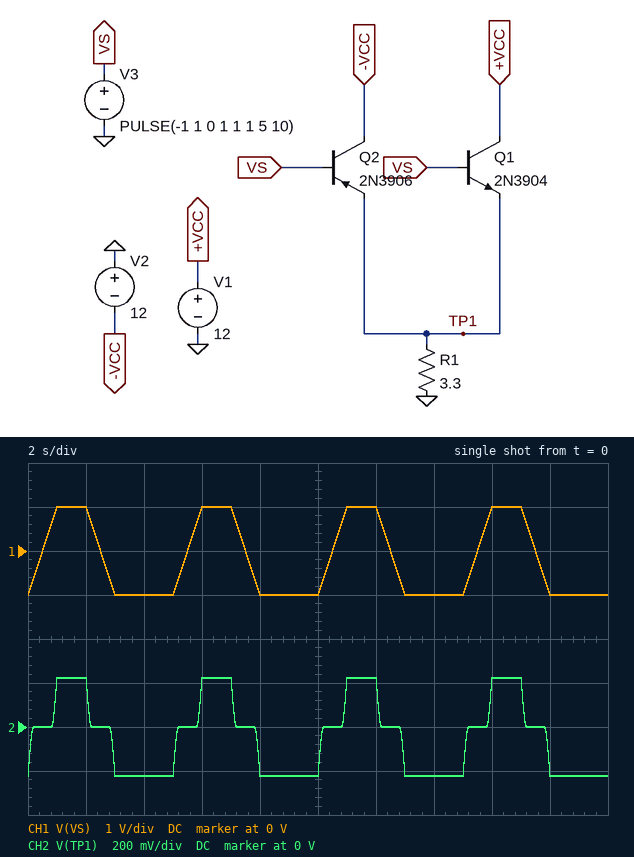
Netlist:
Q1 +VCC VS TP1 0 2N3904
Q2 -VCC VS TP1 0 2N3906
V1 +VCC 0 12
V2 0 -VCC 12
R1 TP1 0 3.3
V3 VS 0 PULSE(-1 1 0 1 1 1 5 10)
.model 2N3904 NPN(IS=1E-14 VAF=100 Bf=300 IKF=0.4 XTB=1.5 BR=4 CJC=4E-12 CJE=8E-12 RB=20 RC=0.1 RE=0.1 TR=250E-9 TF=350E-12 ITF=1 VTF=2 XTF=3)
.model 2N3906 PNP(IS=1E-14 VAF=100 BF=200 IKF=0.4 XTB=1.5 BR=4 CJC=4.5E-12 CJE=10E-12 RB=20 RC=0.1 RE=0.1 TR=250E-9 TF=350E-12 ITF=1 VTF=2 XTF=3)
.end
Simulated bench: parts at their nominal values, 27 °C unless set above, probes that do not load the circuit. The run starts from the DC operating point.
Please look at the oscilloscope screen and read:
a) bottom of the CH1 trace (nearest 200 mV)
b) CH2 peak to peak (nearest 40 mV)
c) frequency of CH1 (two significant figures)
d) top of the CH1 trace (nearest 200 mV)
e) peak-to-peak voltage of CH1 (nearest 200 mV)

-1.0 V
440 mV
200 mHz
1.0 V
2.0 V
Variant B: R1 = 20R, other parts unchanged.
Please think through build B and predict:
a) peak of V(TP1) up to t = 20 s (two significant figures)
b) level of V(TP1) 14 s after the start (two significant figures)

280 mV
-280 mV
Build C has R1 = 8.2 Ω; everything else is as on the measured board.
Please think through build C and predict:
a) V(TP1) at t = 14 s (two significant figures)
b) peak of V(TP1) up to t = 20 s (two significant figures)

-250 mV
250 mV
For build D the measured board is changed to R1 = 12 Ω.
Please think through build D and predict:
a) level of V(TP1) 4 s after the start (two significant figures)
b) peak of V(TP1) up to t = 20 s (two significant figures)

-260 mV
260 mV
